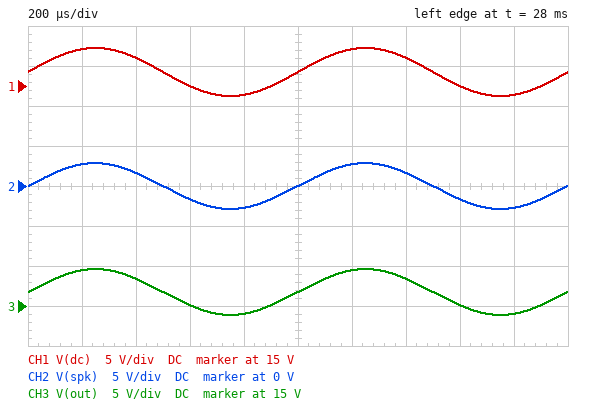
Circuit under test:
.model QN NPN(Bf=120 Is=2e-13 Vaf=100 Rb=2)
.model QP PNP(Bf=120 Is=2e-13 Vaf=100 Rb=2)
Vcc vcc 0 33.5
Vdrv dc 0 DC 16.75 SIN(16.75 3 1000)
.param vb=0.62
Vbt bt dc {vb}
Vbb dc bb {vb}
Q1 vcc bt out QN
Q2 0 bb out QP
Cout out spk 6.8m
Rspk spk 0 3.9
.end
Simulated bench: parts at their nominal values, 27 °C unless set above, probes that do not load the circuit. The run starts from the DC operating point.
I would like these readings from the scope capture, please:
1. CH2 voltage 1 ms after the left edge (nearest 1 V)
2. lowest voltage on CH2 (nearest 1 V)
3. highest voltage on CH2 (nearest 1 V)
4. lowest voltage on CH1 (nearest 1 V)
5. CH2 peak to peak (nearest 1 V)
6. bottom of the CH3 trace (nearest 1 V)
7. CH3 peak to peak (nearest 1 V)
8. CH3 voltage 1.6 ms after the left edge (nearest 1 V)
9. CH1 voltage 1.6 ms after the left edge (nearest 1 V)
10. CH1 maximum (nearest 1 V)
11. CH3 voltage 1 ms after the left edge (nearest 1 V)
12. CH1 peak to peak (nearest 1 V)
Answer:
0 V
-3 V
3 V
14 V
6 V
14 V
6 V
15 V
15 V
20 V
17 V
6 V
